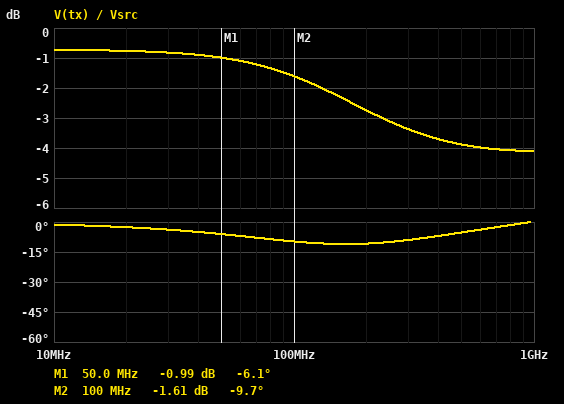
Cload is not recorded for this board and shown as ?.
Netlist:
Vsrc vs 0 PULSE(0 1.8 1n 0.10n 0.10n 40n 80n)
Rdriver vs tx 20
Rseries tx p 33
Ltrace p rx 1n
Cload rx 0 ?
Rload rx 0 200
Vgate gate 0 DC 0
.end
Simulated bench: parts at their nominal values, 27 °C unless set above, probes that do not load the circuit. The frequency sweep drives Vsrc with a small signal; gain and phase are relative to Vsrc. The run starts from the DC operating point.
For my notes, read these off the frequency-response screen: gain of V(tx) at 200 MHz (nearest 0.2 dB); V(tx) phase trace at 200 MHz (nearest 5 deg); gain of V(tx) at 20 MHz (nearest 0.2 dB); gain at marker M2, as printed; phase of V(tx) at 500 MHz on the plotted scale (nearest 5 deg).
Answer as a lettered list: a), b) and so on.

a) -2.8 dB
b) -10 deg
c) -0.8 dB
d) -1.61 dB
e) -5 deg
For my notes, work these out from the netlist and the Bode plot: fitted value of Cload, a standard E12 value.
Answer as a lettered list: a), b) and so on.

a) 27 pF
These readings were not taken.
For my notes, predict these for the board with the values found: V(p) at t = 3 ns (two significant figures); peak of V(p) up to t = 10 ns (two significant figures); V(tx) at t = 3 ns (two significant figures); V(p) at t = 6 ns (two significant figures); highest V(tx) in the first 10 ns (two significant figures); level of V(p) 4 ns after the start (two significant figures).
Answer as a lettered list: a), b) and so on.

a) 1.2 V
b) 1.4 V
c) 1.6 V
d) 1.4 V
e) 1.7 V
f) 1.3 V
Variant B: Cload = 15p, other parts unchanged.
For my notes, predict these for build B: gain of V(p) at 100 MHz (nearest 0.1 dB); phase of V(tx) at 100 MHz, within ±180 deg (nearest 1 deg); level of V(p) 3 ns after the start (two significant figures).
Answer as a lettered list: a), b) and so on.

a) -2.7 dB
b) -7 deg
c) 1.4 V
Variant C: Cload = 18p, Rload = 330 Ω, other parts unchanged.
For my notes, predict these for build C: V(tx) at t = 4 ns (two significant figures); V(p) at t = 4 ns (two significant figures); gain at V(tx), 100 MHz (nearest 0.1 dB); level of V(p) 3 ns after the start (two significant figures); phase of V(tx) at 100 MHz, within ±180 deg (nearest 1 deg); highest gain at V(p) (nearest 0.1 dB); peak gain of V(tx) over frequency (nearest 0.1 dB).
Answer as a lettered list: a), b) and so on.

a) 1.7 V
b) 1.5 V
c) -1.0 dB
d) 1.4 V
e) -9 deg
f) -1.3 dB
g) -0.5 dB
